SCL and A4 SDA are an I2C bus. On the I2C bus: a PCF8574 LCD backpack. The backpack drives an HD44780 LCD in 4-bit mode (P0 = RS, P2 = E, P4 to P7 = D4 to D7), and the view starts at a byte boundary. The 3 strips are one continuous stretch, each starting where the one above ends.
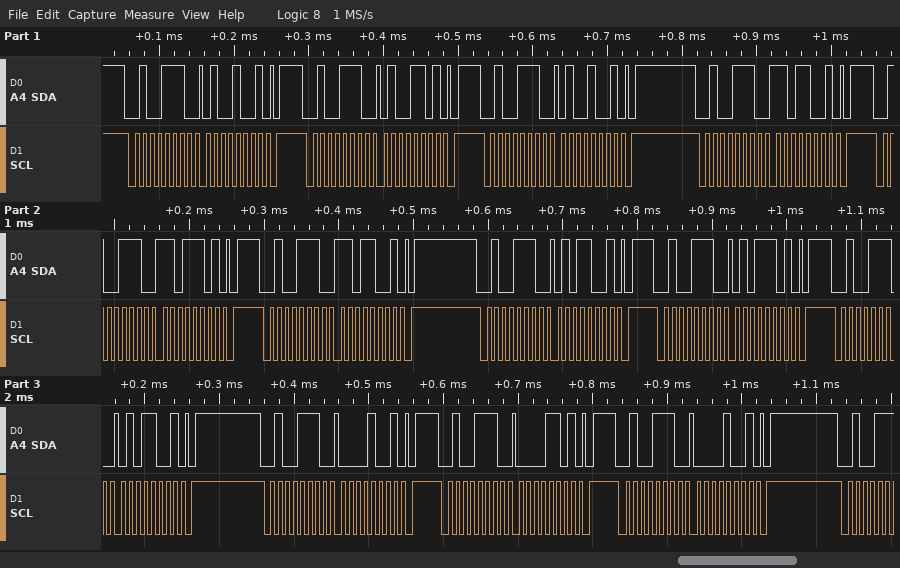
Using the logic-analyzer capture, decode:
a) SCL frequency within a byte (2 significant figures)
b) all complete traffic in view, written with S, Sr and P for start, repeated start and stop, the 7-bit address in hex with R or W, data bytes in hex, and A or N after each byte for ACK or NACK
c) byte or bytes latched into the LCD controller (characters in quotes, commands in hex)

100 kHz
S 27W A 49 A P S 27W A 4D A P S 27W A 49 A P S 27W A D9 A P S 27W A DD A P S 27W A D9 A P S 27W A 59 A P S 27W A 5D A P S 27W A 59 A P S 27W A 09 A P S 27W A 0D A P S 27W A 09 A P
'M' 'P'
